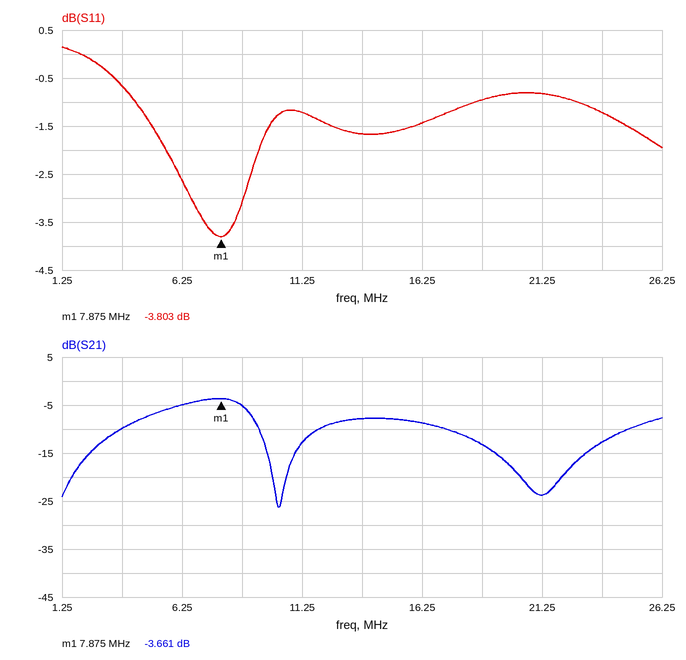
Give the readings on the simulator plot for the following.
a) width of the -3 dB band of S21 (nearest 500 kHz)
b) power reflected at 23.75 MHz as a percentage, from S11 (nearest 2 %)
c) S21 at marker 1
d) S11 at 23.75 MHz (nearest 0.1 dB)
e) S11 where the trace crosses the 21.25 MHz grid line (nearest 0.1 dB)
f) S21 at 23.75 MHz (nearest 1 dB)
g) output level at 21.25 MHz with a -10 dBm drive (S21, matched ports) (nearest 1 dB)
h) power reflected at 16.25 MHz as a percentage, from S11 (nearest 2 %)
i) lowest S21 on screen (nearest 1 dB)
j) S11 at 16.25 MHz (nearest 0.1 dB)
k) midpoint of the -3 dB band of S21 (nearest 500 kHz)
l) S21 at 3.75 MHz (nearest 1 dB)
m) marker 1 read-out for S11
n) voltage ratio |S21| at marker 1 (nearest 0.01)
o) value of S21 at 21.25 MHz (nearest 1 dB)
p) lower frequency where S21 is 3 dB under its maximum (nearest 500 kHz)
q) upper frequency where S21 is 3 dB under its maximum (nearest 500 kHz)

4.0 MHz
76 %
-3.661 dB
-1.2 dB
-0.8 dB
-13 dB
-34 dBm
72 %
-26 dB
-1.4 dB
7.0 MHz
-10 dB
-3.803 dB
0.66
-24 dB
5.0 MHz
9.0 MHz
